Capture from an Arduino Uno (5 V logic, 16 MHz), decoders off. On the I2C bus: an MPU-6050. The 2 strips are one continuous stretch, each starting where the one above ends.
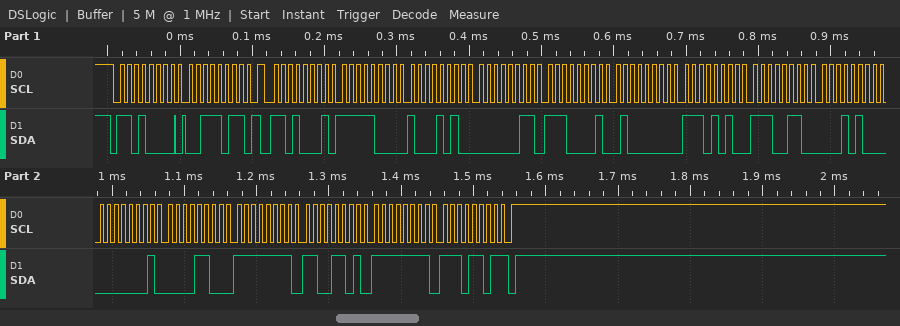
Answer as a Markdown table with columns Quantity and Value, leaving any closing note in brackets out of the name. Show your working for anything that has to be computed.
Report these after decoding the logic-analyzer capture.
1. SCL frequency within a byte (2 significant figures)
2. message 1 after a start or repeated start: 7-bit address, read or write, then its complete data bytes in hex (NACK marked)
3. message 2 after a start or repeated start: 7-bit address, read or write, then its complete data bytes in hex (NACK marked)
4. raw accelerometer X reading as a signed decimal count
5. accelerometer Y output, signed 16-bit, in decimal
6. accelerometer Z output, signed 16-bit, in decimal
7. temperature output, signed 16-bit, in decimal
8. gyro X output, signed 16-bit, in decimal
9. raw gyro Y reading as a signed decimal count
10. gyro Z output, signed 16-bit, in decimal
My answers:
| Quantity | Value |
|---|---|
| SCL frequency within a byte | 100 kHz |
| message 1 after a start or repeated start: 7-bit address, read or write, then its complete data bytes in hex | 0x68 write: 3B |
| message 2 after a start or repeated start: 7-bit address, read or write, then its complete data bytes in hex | 0x68 read: F8 8A 03 E1 40 EA E6 14 01 0C FF CD FF ED NACK |
| raw accelerometer X reading as a signed decimal count | 0xF88A = -1910 |
| accelerometer Y output, signed 16-bit, in decimal | 0x03E1 = 993 |
| accelerometer Z output, signed 16-bit, in decimal | 0x40EA = 16618 |
| temperature output, signed 16-bit, in decimal | 0xE614 = -6636 |
| gyro X output, signed 16-bit, in decimal | 0x010C = 268 |
| raw gyro Y reading as a signed decimal count | 0xFFCD = -51 |
| gyro Z output, signed 16-bit, in decimal | 0xFFED = -19 |
